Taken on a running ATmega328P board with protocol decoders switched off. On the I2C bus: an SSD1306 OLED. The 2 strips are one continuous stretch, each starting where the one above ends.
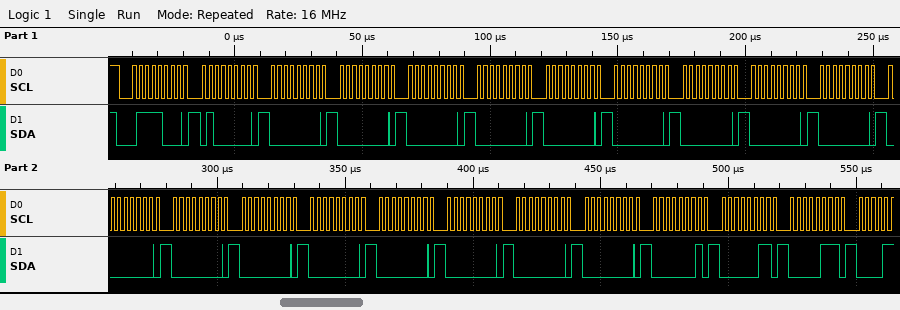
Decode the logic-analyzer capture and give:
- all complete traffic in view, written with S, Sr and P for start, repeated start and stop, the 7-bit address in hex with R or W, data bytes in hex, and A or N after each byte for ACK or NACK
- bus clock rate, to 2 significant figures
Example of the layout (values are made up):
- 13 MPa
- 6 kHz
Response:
- S 3CW A 40 A 00 A 00 A 00 A 00 A 00 A 00 A 00 A 00 A 00 A 00 A 00 A 00 A 00 A 00 A 00 A 00 A 00 A 01 A 03 A 07 A
- 400 kHz
